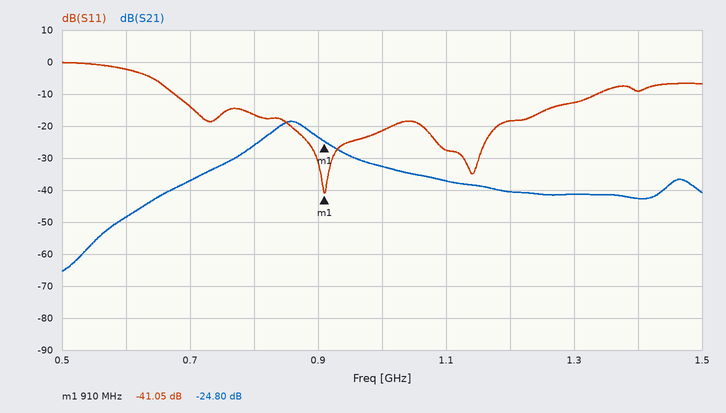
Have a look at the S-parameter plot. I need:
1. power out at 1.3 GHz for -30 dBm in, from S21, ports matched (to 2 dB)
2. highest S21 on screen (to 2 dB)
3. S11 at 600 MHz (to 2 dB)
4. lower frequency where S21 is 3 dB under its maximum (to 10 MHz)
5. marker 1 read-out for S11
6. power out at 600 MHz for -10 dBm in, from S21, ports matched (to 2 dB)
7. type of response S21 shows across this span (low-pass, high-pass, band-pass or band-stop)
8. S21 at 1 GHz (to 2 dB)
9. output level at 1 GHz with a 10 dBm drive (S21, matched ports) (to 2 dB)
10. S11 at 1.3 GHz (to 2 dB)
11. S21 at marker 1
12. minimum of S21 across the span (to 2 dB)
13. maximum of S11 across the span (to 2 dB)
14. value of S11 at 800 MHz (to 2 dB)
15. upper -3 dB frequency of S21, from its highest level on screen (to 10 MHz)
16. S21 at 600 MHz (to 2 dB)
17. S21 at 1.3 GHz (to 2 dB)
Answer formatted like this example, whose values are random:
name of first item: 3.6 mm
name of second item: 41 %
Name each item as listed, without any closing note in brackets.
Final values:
power out at 1.3 GHz for -30 dBm in, from S21, ports matched: -72 dBm
highest S21 on screen: -18 dB
S11 at 600 MHz: -2 dB
lower frequency where S21 is 3 dB under its maximum: 830 MHz
marker 1 read-out for S11: -41.05 dB
power out at 600 MHz for -10 dBm in, from S21, ports matched: -58 dBm
type of response S21 shows across this span: band-pass
S21 at 1 GHz: -32 dB
output level at 1 GHz with a 10 dBm drive (S21, matched ports): -22 dBm
S11 at 1.3 GHz: -12 dB
S21 at marker 1: -24.80 dB
minimum of S21 across the span: -66 dB
maximum of S11 across the span: 0 dB
value of S11 at 800 MHz: -16 dB
upper -3 dB frequency of S21, from its highest level on screen: 890 MHz
S21 at 600 MHz: -48 dB
S21 at 1.3 GHz: -42 dB
